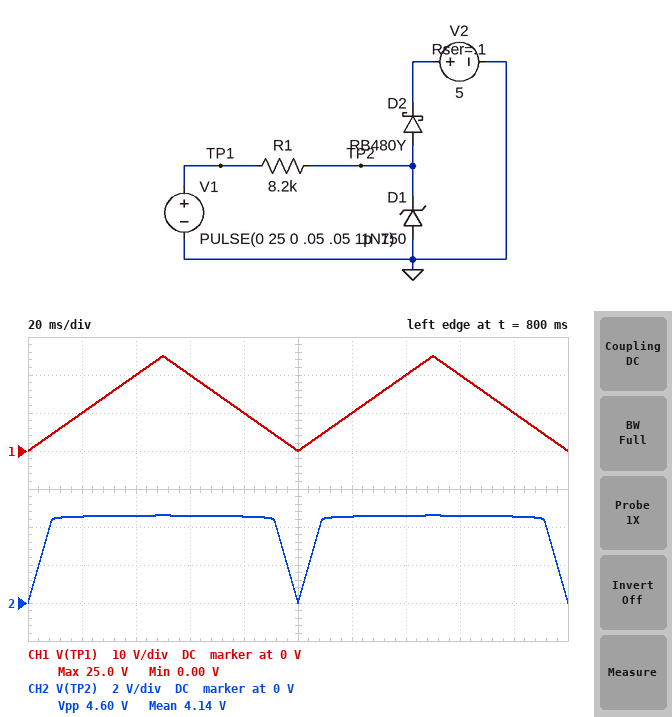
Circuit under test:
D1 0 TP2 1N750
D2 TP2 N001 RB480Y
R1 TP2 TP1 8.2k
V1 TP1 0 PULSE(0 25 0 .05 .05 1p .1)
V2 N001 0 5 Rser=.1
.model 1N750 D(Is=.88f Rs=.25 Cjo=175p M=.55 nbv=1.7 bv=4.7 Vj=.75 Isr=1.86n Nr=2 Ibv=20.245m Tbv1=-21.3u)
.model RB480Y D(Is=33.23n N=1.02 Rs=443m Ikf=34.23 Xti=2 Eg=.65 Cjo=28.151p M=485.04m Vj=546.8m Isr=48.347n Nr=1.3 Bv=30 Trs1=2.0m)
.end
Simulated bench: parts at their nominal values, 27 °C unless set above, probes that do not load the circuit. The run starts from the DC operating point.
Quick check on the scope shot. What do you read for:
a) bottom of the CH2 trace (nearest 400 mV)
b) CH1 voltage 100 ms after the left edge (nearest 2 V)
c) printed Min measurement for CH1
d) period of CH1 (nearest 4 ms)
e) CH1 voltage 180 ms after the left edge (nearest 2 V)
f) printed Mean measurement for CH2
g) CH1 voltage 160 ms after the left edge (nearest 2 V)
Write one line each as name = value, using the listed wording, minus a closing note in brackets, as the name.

bottom of the CH2 trace = 0 V
CH1 voltage 100 ms after the left edge = 0 V
printed Min measurement for CH1 = 0.00 V
period of CH1 = 100 ms
CH1 voltage 180 ms after the left edge = 10 V
printed Mean measurement for CH2 = 4.14 V
CH1 voltage 160 ms after the left edge = 20 V
